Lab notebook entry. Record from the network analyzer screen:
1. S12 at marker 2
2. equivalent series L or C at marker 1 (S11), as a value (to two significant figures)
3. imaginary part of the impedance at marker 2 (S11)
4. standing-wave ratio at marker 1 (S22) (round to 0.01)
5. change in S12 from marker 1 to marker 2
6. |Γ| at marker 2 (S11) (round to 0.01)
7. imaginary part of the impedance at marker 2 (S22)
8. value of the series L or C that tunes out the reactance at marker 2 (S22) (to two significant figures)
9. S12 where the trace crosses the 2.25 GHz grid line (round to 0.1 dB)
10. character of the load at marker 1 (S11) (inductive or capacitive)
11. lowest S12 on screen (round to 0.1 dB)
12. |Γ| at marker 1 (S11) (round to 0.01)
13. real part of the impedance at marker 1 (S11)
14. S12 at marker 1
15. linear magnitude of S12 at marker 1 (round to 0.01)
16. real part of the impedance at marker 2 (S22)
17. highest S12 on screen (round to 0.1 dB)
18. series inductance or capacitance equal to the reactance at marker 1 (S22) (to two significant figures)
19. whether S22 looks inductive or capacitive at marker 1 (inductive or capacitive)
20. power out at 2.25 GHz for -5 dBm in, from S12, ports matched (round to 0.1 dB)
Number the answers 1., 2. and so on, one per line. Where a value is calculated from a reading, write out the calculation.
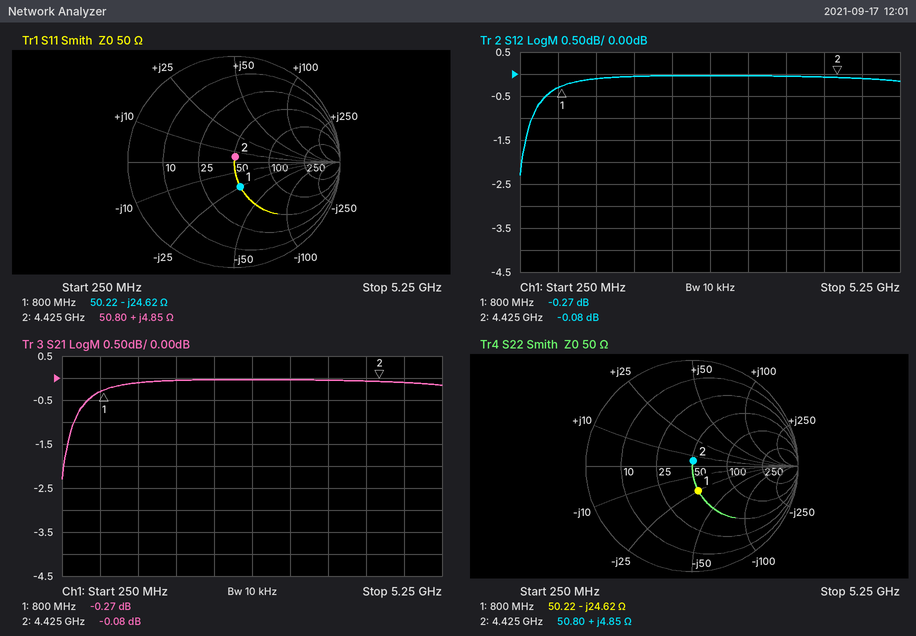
1. -0.08 dB
2. C = 1/(2π × 800 MHz × 24.62 Ω) ≈ 8.1 pF
3. +4.85 Ω
4. 1.63
5. -0.08 − (-0.27) = 0.19 dB
6. 0.05
7. +4.85 Ω
8. C = 1/(2π × 4.425 GHz × 4.85 Ω) ≈ 7.4 pF
9. 0.0 dB
10. capacitive
11. -2.3 dB
12. 0.24
13. 50.22 Ω
14. -0.27 dB
15. 10^(-0.27/20) ≈ 0.97
16. 50.80 Ω
17. 0.0 dB
18. C = 1/(2π × 800 MHz × 24.62 Ω) ≈ 8.1 pF
19. capacitive
20. -5 dBm + (0.0 dB) = -5.0 dBm
